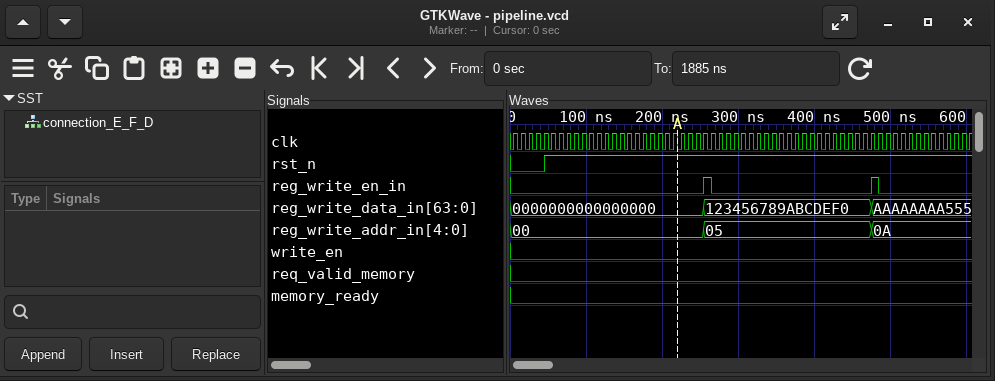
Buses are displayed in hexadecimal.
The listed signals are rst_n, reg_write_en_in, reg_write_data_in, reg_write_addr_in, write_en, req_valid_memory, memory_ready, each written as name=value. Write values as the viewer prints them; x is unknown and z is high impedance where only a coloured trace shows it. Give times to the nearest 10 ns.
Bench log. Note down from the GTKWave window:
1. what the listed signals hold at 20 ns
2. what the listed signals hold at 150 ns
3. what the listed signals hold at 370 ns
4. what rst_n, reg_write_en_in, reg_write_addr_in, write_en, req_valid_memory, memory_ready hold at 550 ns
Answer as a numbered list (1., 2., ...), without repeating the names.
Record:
1. rst_n=0, reg_write_en_in=0, reg_write_data_in=0000000000000000, reg_write_addr_in=00, write_en=0, req_valid_memory=0, memory_ready=0
2. rst_n=1, reg_write_en_in=0, reg_write_data_in=0000000000000000, reg_write_addr_in=00, write_en=0, req_valid_memory=0, memory_ready=0
3. rst_n=1, reg_write_en_in=0, reg_write_data_in=123456789ABCDEF0, reg_write_addr_in=05, write_en=0, req_valid_memory=0, memory_ready=0
4. rst_n=1, reg_write_en_in=0, reg_write_addr_in=0A, write_en=0, req_valid_memory=0, memory_ready=0
